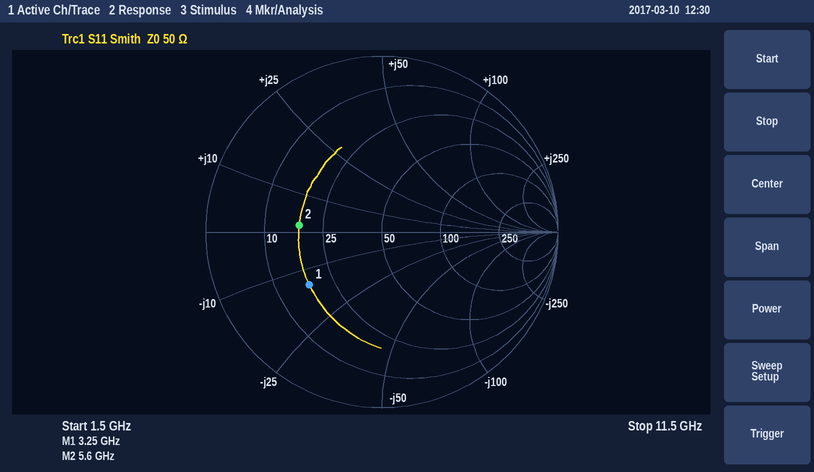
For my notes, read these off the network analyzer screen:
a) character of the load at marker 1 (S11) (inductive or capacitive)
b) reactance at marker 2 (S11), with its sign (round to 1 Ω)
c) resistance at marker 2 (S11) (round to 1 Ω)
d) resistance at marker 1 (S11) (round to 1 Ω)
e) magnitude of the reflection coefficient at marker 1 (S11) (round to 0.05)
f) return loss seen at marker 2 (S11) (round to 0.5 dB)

capacitive
+2 Ω
18 Ω
18 Ω
0.50
6.5 dB
